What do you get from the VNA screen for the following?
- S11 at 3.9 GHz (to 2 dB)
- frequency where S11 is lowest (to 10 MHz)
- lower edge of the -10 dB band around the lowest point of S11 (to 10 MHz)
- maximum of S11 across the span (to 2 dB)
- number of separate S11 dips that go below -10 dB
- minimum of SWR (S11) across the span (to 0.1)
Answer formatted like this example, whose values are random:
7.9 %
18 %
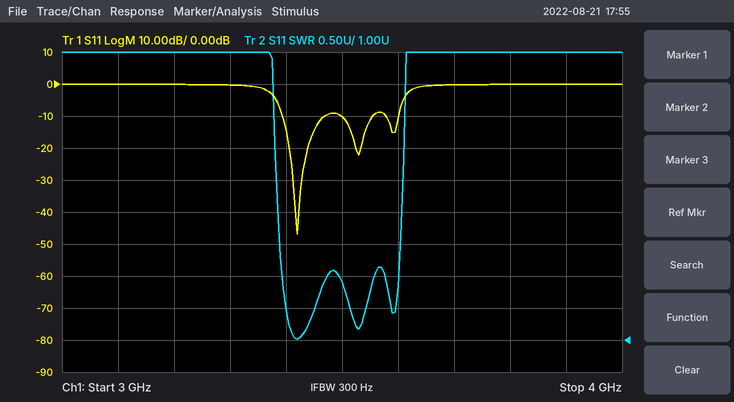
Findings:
0 dB
3.42 GHz
3.39 GHz
0 dB
3
1.0
